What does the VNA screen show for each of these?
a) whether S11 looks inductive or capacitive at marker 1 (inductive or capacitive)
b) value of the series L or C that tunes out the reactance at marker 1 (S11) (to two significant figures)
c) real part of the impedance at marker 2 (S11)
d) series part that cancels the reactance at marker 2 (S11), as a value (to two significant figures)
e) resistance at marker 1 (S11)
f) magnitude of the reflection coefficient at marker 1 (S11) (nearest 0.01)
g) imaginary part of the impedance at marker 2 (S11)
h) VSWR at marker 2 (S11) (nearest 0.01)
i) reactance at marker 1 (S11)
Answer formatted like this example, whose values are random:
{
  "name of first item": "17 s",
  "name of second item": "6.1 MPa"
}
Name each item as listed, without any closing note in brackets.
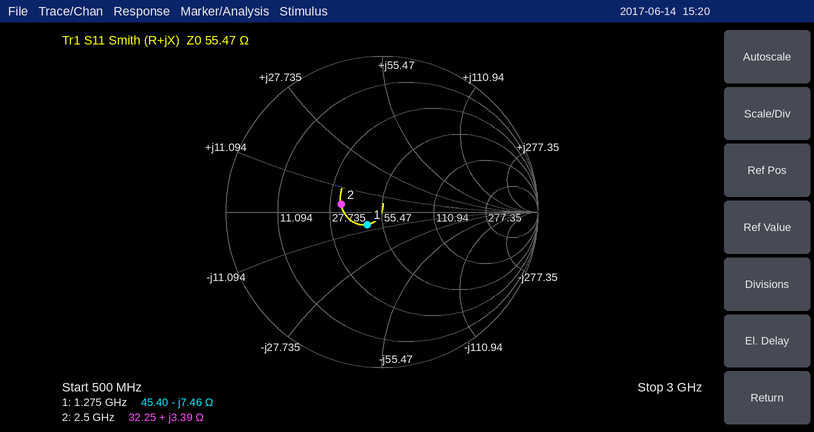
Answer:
{
  "whether S11 looks inductive or capacitive at marker 1": "capacitive",
  "value of the series L or C that tunes out the reactance at marker 1 (S11)": "930 pH",
  "real part of the impedance at marker 2": "32.25 Ω",
  "series part that cancels the reactance at marker 2 (S11), as a value": "19 pF",
  "resistance at marker 1": "45.40 Ω",
  "magnitude of the reflection coefficient at marker 1 (S11)": "0.12",
  "imaginary part of the impedance at marker 2": "+3.39 Ω",
  "VSWR at marker 2 (S11)": "1.73",
  "reactance at marker 1": "-7.46 Ω"
}
